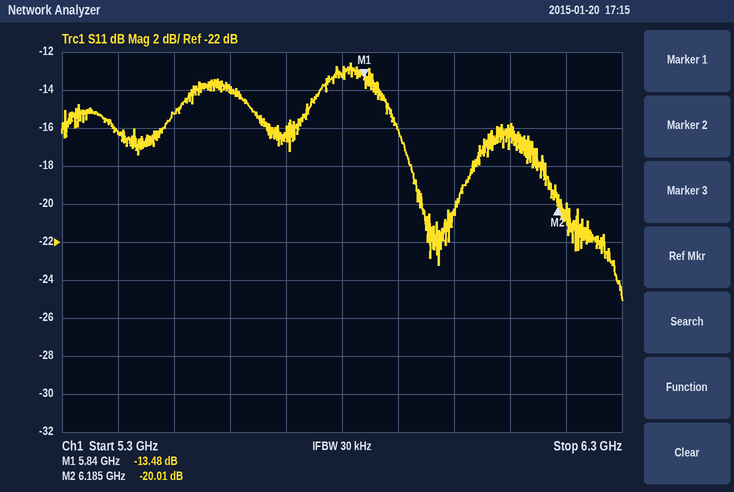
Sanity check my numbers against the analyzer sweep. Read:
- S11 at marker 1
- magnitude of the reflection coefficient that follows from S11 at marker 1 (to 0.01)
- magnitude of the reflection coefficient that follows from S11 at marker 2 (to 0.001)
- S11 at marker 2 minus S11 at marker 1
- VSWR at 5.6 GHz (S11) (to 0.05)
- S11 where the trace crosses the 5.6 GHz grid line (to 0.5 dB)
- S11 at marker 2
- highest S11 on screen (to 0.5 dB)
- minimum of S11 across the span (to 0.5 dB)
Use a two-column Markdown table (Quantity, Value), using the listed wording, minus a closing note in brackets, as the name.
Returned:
| Quantity | Value |
|---|---|
| S11 at marker 1 | -13.48 dB |
| magnitude of the reflection coefficient that follows from S11 at marker 1 | 0.21 |
| magnitude of the reflection coefficient that follows from S11 at marker 2 | 0.100 |
| S11 at marker 2 minus S11 at marker 1 | -6.53 dB |
| VSWR at 5.6 GHz (S11) | 1.50 |
| S11 where the trace crosses the 5.6 GHz grid line | -14.0 dB |
| S11 at marker 2 | -20.01 dB |
| highest S11 on screen | -12.5 dB |
| minimum of S11 across the span | -25.0 dB |
